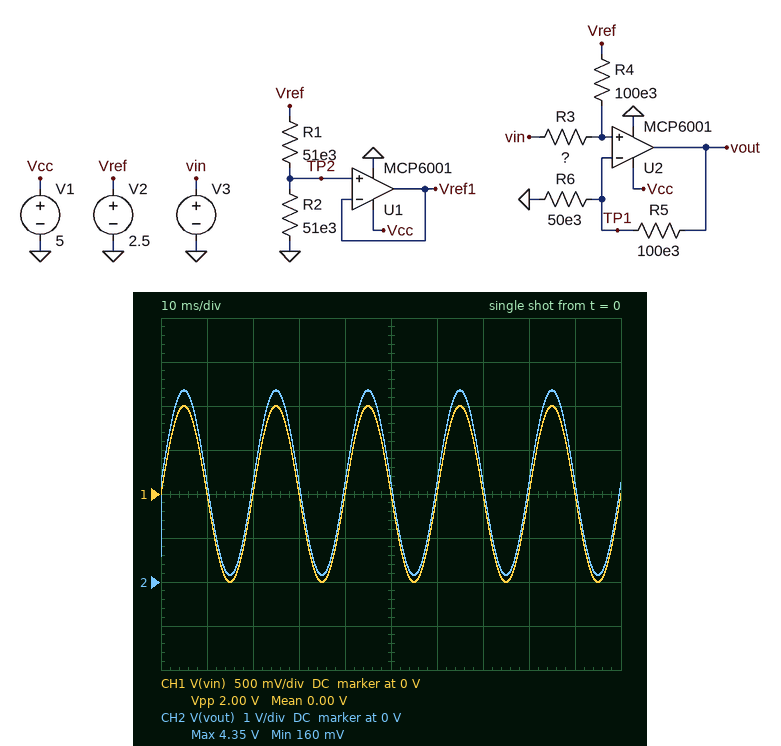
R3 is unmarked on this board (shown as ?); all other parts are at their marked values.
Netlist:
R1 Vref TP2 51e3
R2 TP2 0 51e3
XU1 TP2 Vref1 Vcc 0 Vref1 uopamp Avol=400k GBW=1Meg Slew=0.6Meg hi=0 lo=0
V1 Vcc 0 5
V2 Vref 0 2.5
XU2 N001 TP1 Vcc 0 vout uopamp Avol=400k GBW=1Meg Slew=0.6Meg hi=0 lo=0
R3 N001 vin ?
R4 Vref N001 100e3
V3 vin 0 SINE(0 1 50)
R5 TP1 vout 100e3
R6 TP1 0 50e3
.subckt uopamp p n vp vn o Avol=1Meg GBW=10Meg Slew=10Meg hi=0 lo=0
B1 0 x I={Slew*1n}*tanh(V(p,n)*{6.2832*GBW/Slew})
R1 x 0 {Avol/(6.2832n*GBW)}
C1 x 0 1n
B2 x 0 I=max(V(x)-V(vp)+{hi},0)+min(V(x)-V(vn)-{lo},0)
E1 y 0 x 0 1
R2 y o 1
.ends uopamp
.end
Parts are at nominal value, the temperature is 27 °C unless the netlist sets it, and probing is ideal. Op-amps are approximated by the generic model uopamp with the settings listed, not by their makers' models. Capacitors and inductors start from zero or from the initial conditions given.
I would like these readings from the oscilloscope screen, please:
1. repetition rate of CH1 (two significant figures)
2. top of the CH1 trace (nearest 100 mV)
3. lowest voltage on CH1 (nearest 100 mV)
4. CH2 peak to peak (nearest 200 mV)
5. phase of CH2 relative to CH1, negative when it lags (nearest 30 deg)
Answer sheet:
50 Hz
1.0 V
-1.0 V
4.2 V
0 deg
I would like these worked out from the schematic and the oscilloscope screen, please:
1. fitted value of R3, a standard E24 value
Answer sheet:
43 kΩ
